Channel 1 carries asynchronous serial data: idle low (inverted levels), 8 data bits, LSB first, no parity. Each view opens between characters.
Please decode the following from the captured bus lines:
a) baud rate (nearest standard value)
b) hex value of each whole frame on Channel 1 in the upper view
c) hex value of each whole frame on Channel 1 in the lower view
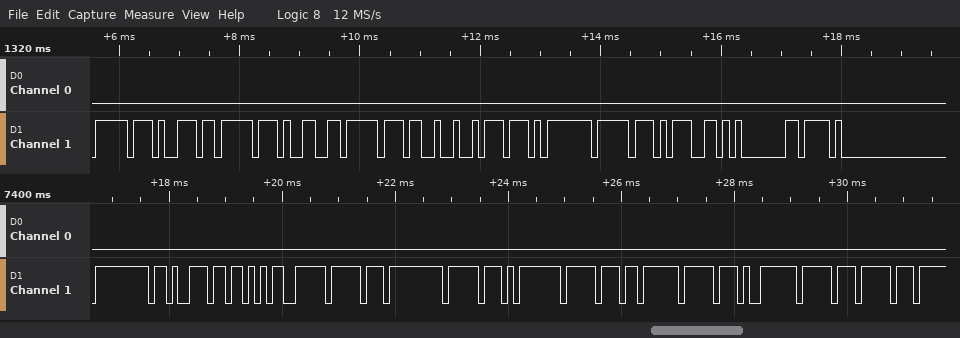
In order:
9600 baud
10, 23, 10, 33, 10, B6, 11, 01, 10, 31, FD, 42
00, 1A, 52, 06, 10, 00, 10, 01, 10, 02, 10, 03, 10, 10
